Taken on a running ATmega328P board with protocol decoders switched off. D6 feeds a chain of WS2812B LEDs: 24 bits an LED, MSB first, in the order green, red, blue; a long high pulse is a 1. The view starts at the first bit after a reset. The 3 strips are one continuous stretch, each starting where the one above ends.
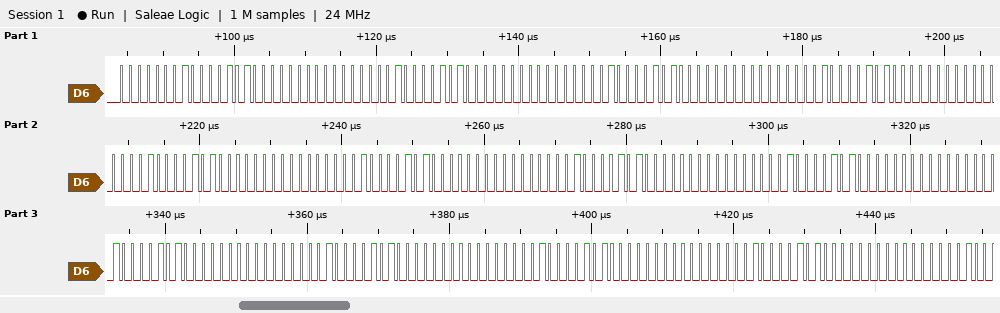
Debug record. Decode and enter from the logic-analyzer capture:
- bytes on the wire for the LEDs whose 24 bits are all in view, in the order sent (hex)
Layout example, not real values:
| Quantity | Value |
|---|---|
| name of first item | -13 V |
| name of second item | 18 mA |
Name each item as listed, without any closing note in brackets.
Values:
| Quantity | Value |
|---|---|
| bytes on the wire for the LEDs whose 24 bits are all in view, in the order sent | 01 0A 00 01 0A 00 01 0A 00 01 0A 00 01 0A 00 01 0A 00 01 0A 00 01 0A 00 01 0A 00 01 0A 00 01 0A 00 01 0A 00 |
